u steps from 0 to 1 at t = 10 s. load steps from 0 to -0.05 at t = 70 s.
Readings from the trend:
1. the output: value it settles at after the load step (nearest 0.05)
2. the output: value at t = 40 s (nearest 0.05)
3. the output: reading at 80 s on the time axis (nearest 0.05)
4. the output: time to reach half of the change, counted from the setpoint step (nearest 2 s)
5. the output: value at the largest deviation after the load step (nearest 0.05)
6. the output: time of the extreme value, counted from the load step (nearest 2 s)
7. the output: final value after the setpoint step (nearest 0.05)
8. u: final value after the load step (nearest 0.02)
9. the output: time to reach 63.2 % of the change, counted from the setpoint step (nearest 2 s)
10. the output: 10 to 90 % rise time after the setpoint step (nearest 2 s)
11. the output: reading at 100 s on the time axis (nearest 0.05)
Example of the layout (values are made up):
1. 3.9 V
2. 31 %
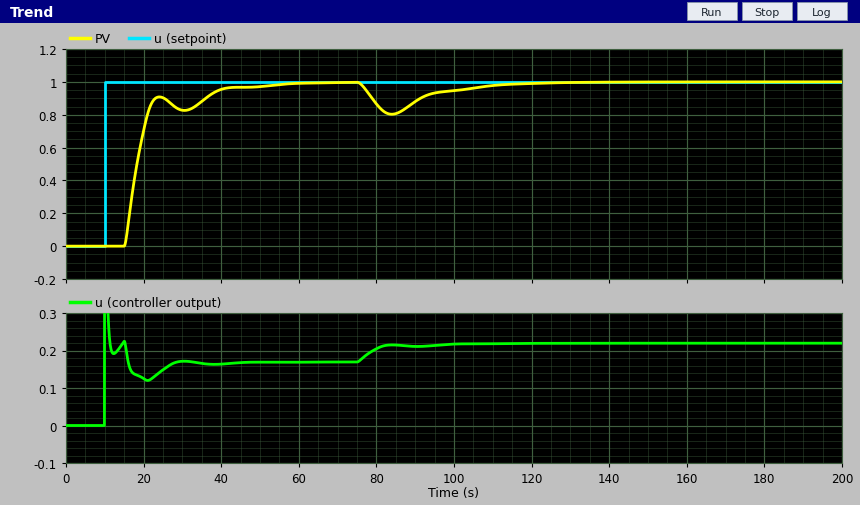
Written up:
1. 1.00
2. 0.95
3. 0.85
4. 8 s
5. 0.80
6. 14 s
7. 1.00
8. 0.22
9. 10 s
10. 8 s
11. 0.95
